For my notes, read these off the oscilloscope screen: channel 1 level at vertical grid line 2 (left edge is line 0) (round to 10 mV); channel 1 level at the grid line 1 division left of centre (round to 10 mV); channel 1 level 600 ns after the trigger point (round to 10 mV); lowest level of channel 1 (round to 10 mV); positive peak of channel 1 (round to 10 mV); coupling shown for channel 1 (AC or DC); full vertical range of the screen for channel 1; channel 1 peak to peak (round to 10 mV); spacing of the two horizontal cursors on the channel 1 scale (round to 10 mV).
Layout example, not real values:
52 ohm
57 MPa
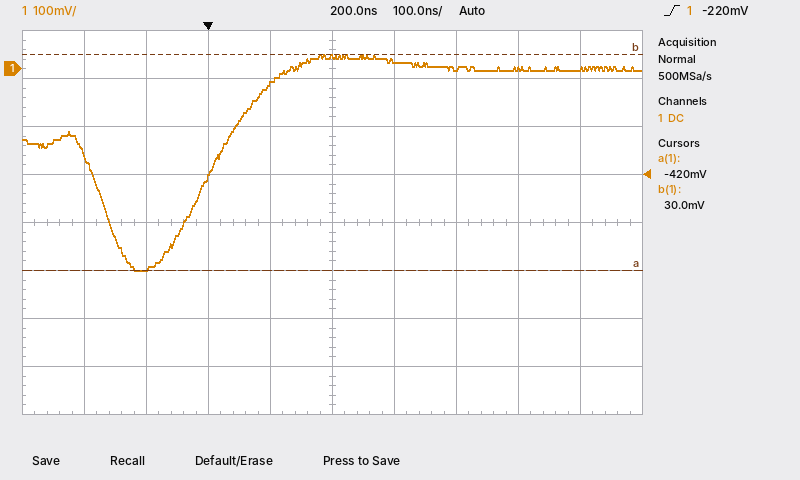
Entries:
-420 mV
-30 mV
0 mV
-420 mV
30 mV
DC
800 mV
450 mV
450 mV
